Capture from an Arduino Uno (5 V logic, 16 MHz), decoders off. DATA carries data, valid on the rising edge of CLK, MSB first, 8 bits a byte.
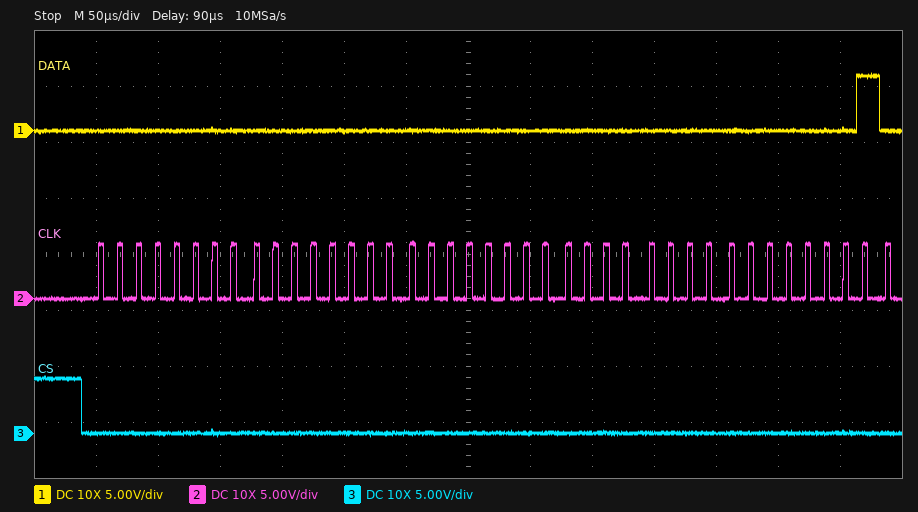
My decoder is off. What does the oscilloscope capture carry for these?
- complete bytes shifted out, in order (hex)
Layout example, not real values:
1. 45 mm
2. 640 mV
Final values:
1. 00 00 00 00 01
